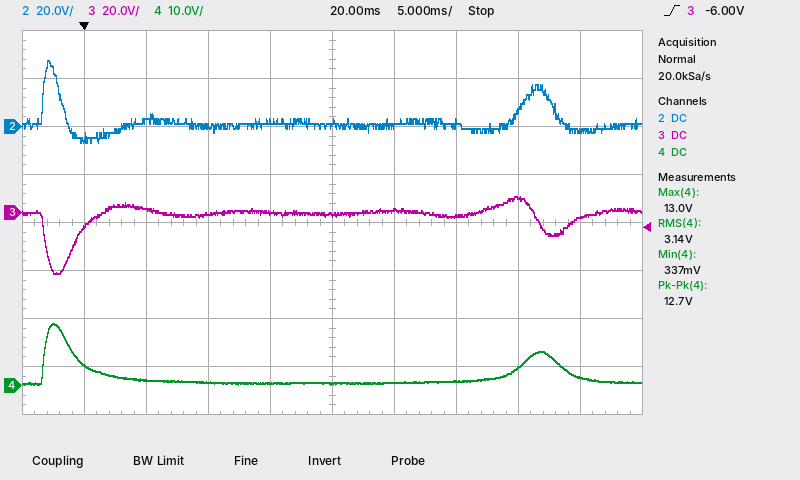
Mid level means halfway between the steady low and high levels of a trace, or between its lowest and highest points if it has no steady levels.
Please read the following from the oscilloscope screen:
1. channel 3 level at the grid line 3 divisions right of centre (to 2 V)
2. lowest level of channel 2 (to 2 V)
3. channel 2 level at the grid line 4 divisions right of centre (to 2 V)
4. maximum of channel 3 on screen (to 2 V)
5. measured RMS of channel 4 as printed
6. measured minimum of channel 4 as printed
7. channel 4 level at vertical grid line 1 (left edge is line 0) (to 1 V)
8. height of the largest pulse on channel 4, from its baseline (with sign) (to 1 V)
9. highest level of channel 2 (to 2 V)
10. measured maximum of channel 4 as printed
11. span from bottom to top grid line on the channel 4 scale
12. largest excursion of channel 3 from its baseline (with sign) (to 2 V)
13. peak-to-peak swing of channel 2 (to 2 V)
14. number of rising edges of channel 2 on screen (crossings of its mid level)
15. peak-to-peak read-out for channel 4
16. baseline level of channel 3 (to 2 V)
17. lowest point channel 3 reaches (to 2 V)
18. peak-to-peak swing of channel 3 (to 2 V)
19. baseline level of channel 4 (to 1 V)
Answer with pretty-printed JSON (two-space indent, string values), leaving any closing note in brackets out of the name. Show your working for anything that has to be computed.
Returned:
{
  "channel 3 level at the grid line 3 divisions right of centre": "6 V",
  "lowest level of channel 2": "-6 V",
  "channel 2 level at the grid line 4 divisions right of centre": "-2 V",
  "maximum of channel 3 on screen": "6 V",
  "measured RMS of channel 4 as printed": "3.14 V",
  "measured minimum of channel 4 as printed": "337 mV",
  "channel 4 level at vertical grid line 1 (left edge is line 0)": "4 V",
  "height of the largest pulse on channel 4, from its baseline (with sign)": "+12 V",
  "highest level of channel 2": "28 V",
  "measured maximum of channel 4 as printed": "13.0 V",
  "span from bottom to top grid line on the channel 4 scale": "80 V",
  "largest excursion of channel 3 from its baseline (with sign)": "-26 V − (0 V) = -26 V",
  "peak-to-peak swing of channel 2": "28 V − (-6 V) = 34 V",
  "number of rising edges of channel 2 on screen": "2",
  "peak-to-peak read-out for channel 4": "12.7 V",
  "baseline level of channel 3": "0 V",
  "lowest point channel 3 reaches": "-26 V",
  "peak-to-peak swing of channel 3": "6 V − (-26 V) = 32 V",
  "baseline level of channel 4": "1 V"
}
